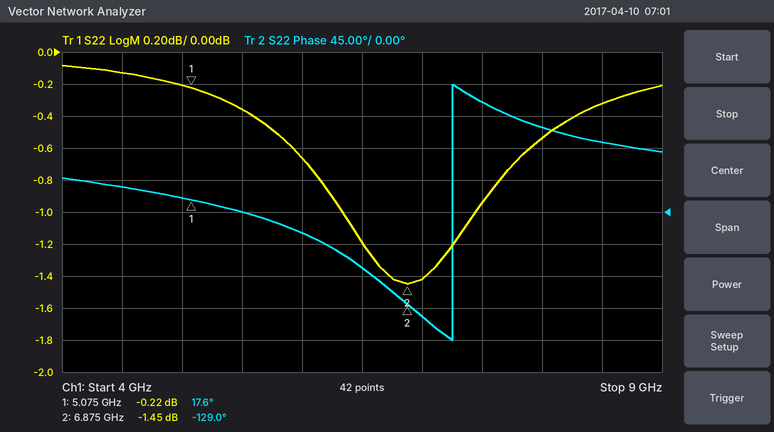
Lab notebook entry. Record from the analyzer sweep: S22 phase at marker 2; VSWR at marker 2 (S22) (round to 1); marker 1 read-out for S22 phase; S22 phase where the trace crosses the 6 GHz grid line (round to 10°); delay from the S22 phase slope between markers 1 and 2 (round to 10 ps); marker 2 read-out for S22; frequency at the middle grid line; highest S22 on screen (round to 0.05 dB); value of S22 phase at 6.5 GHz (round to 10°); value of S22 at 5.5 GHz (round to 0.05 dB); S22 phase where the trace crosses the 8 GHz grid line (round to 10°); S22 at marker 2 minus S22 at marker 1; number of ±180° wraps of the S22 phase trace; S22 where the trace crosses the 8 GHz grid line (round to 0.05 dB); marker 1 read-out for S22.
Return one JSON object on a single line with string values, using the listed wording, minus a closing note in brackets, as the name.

{"S22 phase at marker 2": "-129.0°", "VSWR at marker 2 (S22)": "12", "marker 1 read-out for S22 phase": "17.6°", "S22 phase where the trace crosses the 6 GHz grid line": "-30°", "delay from the S22 phase slope between markers 1 and 2": "230 ps", "marker 2 read-out for S22": "-1.45 dB", "frequency at the middle grid line": "6.5 GHz", "highest S22 on screen": "-0.10 dB", "value of S22 phase at 6.5 GHz": "-80°", "value of S22 at 5.5 GHz": "-0.35 dB", "S22 phase where the trace crosses the 8 GHz grid line": "120°", "S22 at marker 2 minus S22 at marker 1": "-1.23 dB", "number of ±180° wraps of the S22 phase trace": "1", "S22 where the trace crosses the 8 GHz grid line": "-0.55 dB", "marker 1 read-out for S22": "-0.22 dB"}
